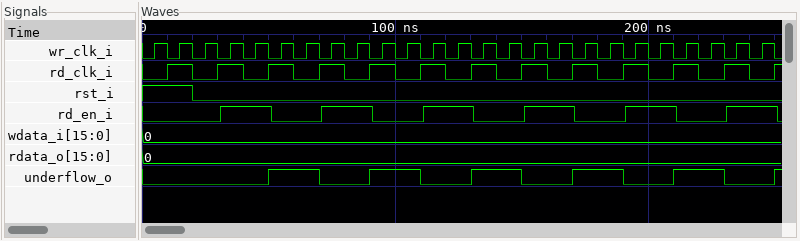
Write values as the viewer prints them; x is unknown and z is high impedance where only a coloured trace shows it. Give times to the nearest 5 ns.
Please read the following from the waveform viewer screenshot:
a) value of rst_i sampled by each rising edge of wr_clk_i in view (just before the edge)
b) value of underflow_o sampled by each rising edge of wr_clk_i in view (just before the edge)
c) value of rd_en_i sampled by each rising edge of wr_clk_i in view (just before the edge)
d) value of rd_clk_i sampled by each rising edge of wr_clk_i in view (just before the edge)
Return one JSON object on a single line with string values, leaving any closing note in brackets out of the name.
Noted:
{"value of rst_i sampled by each rising edge of wr_clk_i in view": "1 1 0 0 0 0 0 0 0 0 0 0 0 0 0 0 0 0 0 0 0 0 0 0 0", "value of underflow_o sampled by each rising edge of wr_clk_i in view": "0 0 0 0 0 1 1 0 0 1 1 0 0 1 1 0 0 1 1 0 0 1 1 0 0", "value of rd_en_i sampled by each rising edge of wr_clk_i in view": "0 0 0 1 1 0 0 1 1 0 0 1 1 0 0 1 1 0 0 1 1 0 0 1 1", "value of rd_clk_i sampled by each rising edge of wr_clk_i in view": "0 1 0 1 0 1 0 1 0 1 0 1 0 1 0 1 0 1 0 1 0 1 0 1 0"}
